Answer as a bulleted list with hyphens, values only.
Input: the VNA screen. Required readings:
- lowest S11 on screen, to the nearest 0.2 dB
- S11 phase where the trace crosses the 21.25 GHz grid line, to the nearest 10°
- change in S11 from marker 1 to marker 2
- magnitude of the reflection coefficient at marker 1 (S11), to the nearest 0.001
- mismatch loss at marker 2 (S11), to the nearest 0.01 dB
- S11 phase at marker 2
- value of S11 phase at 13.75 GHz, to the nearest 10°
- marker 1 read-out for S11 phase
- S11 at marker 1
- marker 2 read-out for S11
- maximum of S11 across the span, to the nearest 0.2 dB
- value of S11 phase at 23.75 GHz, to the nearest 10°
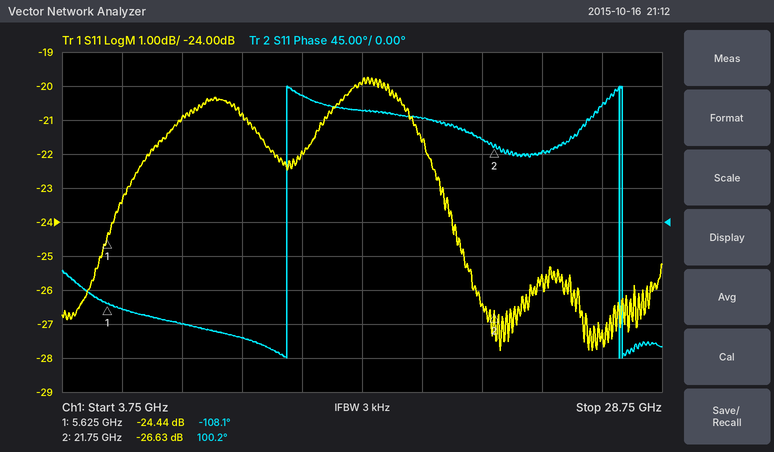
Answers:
- -27.8 dB
- 110°
- -2.19 dB
- 0.060
- 0.01 dB
- 100.2°
- 170°
- -108.1°
- -24.44 dB
- -26.63 dB
- -19.8 dB
- 90°
